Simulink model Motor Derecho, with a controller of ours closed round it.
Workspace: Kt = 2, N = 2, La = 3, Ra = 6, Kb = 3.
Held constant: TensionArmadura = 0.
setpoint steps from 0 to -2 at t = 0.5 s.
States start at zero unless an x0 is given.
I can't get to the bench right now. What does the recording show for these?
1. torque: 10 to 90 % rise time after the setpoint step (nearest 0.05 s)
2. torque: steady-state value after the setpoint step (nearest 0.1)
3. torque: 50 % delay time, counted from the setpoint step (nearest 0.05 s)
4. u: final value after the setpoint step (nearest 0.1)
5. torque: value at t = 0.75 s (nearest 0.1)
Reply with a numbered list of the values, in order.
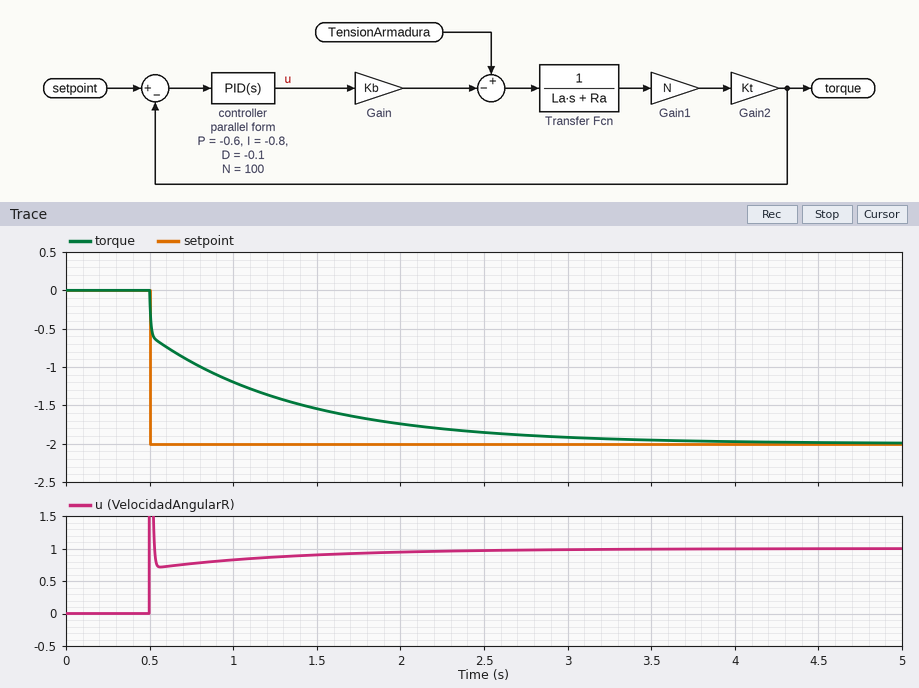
1. 1.70 s
2. -2.0
3. 0.30 s
4. 1.0
5. -0.9
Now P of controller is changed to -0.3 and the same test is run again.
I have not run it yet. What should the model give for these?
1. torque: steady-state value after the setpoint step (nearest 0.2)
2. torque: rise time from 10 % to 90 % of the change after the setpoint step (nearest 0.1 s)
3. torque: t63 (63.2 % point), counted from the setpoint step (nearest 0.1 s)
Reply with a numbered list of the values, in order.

1. -2.0
2. 1.6 s
3. 0.8 s
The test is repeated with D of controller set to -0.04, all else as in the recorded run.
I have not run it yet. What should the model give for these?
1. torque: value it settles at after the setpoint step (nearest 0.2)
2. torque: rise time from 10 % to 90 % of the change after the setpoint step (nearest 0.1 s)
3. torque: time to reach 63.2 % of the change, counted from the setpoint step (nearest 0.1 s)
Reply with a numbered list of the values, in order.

1. -2.0
2. 1.6 s
3. 0.5 s
